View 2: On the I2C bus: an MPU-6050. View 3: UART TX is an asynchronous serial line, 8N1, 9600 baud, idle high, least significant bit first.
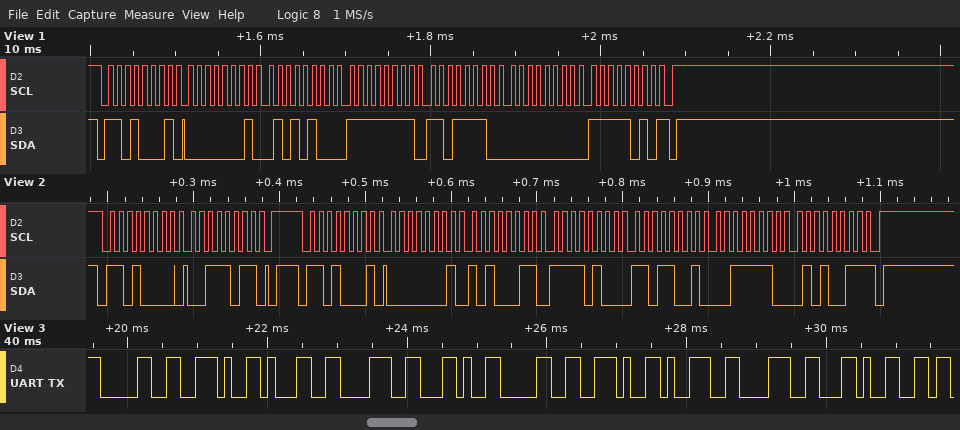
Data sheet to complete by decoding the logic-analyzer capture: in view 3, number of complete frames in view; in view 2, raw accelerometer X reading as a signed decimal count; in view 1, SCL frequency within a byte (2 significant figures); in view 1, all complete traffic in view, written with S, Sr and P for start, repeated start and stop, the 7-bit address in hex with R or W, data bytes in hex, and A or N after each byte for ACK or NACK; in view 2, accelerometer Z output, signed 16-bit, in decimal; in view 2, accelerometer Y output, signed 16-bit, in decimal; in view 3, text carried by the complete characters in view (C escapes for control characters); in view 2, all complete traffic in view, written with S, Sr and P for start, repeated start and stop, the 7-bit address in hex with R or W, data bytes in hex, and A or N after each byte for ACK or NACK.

10
419
100 kHz
S 68R A 01 A 54 A FF A DE A 00 A FA N P
15955
-2855
"0.18,0.98,"
S 68W A 3B A P S 68R A 01 A A3 A F4 A D9 A 3E A 53 N P
